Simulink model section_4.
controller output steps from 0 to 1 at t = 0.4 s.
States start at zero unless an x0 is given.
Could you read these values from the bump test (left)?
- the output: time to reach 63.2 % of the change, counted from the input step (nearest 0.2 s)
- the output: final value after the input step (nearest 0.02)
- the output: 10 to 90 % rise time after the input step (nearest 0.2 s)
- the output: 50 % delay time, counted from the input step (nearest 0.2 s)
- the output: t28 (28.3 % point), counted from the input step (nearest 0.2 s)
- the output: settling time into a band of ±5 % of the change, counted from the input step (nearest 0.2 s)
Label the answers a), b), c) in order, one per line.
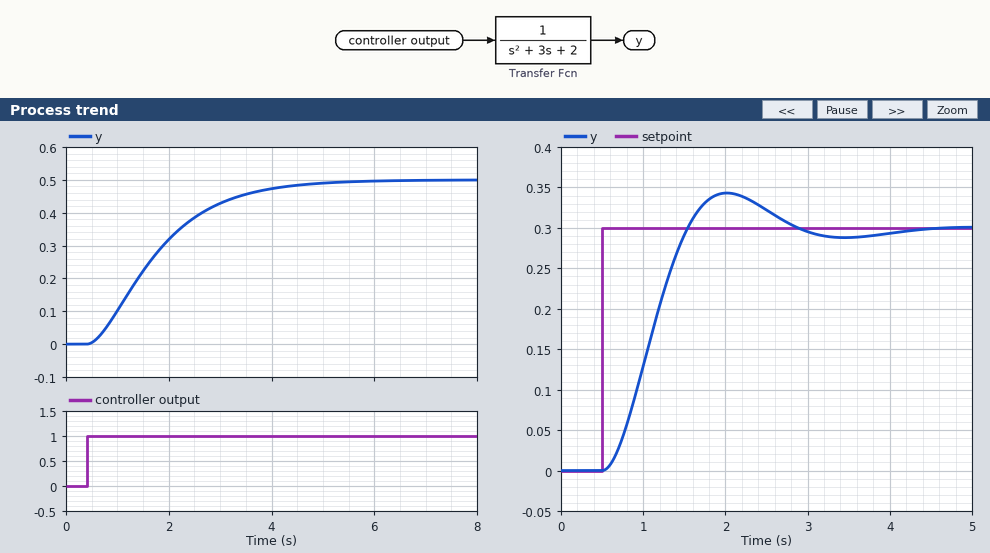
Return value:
a) 1.6 s
b) 0.50
c) 2.6 s
d) 1.2 s
e) 0.8 s
f) 3.6 s
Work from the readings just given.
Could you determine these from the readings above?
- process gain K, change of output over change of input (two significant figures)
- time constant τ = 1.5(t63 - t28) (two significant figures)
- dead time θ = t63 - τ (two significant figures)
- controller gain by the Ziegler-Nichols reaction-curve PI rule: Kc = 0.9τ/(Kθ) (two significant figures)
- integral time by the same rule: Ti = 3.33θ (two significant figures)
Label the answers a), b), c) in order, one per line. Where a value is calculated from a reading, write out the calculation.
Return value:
a) (0.5 - 0) / 1 = 0.50
b) 1.5 × (1.6 - 0.8) = 1.2 s
c) 1.6 - 1.2 = 0.40 s
d) 0.9 × 1.2 / (0.5 × 0.4) = 5.4
e) 3.33 × 0.4 = 1.3 s
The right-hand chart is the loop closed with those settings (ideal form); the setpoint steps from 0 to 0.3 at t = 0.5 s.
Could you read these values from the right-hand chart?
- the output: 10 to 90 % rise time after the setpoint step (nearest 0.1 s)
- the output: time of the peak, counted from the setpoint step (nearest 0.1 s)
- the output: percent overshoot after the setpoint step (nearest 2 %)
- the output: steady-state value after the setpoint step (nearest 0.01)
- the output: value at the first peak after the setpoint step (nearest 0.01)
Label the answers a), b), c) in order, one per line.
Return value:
a) 0.7 s
b) 1.5 s
c) 14 %
d) 0.30
e) 0.34
